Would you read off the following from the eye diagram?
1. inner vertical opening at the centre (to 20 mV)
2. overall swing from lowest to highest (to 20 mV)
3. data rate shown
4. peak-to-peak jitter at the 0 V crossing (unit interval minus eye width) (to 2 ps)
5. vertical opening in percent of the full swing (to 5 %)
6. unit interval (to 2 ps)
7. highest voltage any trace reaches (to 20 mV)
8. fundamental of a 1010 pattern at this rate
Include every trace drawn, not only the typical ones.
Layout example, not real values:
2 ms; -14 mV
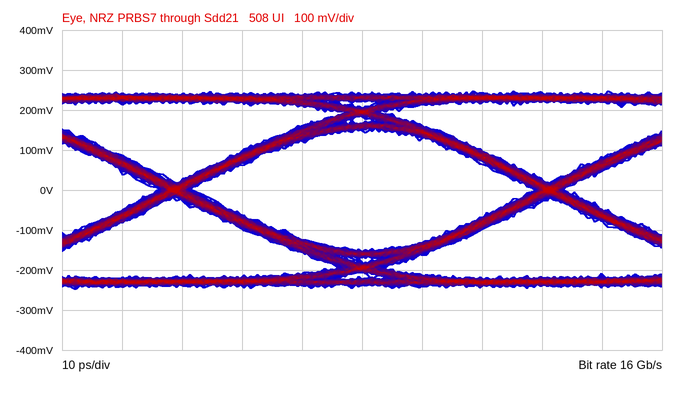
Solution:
300 mV; 500 mV; 16 Gb/s; 6 ps; 60 %; 62 ps; 240 mV; 8 GHz
